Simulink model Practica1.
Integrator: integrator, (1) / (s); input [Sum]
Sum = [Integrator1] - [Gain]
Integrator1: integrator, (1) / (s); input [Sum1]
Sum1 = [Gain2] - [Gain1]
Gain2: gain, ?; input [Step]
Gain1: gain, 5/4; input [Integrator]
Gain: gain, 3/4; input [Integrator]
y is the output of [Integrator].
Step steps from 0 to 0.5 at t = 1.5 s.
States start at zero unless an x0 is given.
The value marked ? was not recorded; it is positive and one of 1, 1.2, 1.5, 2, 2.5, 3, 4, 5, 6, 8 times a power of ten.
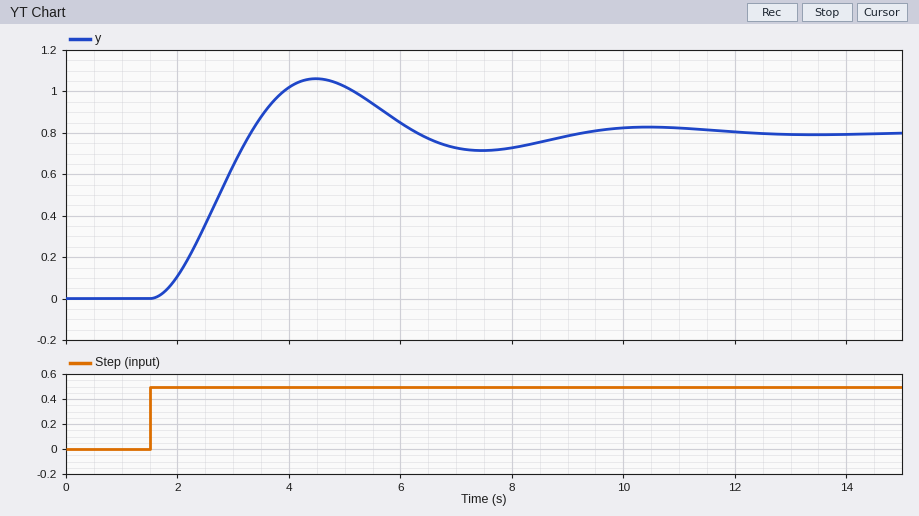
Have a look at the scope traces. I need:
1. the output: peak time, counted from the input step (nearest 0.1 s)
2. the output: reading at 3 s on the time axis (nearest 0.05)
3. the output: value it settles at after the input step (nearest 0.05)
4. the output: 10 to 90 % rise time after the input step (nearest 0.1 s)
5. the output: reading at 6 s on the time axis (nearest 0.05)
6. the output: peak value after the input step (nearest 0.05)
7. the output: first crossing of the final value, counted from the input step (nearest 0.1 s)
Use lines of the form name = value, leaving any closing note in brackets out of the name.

the output: peak time, counted from the input step = 3.0 s
the output: reading at 3 s on the time axis = 0.65
the output: value it settles at after the input step = 0.80
the output: 10 to 90 % rise time after the input step = 1.2 s
the output: reading at 6 s on the time axis = 0.85
the output: peak value after the input step = 1.05
the output: first crossing of the final value, counted from the input step = 1.8 s
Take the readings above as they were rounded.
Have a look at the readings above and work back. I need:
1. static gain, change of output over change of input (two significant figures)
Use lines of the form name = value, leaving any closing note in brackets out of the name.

static gain, change of output over change of input = 1.6
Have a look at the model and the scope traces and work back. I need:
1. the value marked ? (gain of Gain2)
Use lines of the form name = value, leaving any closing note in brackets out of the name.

the value marked ? = 2
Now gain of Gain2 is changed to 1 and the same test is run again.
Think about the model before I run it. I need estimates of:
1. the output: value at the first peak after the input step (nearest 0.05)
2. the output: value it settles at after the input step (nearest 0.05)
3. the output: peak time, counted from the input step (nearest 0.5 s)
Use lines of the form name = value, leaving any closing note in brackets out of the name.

the output: value at the first peak after the input step = 0.55
the output: value it settles at after the input step = 0.40
the output: peak time, counted from the input step = 3.0 s
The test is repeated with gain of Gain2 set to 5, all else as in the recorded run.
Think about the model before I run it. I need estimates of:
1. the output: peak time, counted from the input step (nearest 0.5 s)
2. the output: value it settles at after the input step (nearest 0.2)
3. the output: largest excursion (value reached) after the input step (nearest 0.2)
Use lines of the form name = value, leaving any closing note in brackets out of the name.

the output: peak time, counted from the input step = 3.0 s
the output: value it settles at after the input step = 2.0
the output: largest excursion (value reached) after the input step = 2.6
